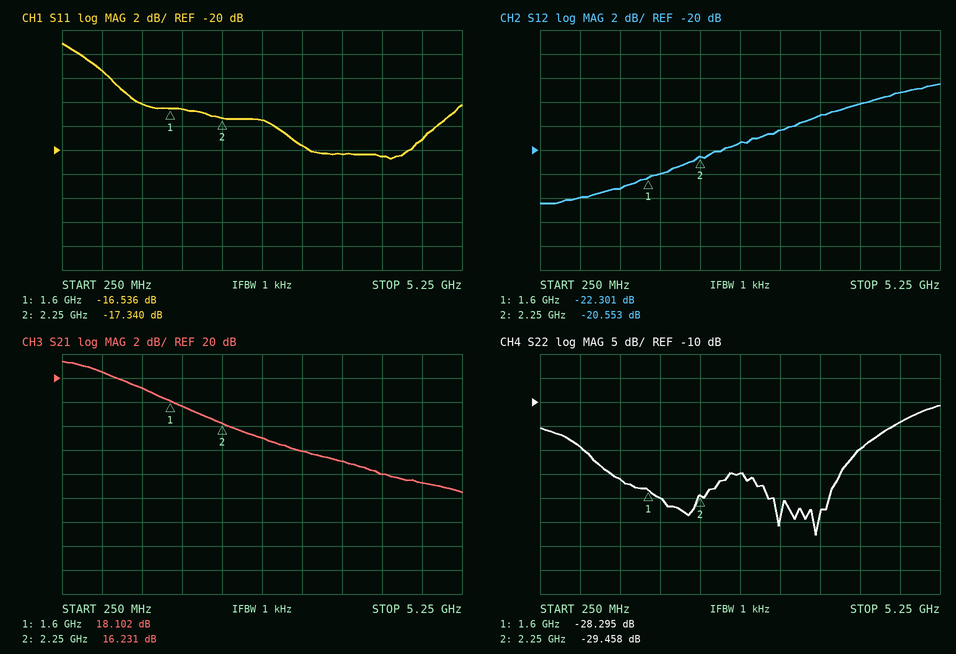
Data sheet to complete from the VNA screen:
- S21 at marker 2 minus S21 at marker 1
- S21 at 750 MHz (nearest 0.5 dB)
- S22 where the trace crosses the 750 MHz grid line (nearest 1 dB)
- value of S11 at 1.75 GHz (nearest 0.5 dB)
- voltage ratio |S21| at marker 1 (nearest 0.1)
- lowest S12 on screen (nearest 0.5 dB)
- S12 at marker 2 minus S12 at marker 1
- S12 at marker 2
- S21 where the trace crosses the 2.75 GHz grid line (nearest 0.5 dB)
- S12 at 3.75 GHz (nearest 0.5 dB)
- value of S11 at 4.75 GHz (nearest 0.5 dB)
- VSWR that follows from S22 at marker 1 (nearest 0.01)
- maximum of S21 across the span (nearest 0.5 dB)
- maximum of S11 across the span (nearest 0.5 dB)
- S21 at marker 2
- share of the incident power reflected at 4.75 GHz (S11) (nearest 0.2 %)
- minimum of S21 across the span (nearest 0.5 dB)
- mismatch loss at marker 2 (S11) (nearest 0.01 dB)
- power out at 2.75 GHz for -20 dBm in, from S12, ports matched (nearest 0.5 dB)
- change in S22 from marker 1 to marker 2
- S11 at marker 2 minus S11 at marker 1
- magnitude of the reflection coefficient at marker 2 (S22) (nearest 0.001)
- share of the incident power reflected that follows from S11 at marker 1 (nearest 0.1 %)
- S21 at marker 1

-1.871 dB
20.5 dB
-19 dB
-16.5 dB
8.0
-24.5 dB
1.748 dB
-20.553 dB
15.0 dB
-17.0 dB
-19.0 dB
1.08
21.5 dB
-11.0 dB
16.231 dB
1.2 %
10.5 dB
0.08 dB
-39.5 dBm
-1.163 dB
-0.804 dB
0.034
2.2 %
18.102 dB
